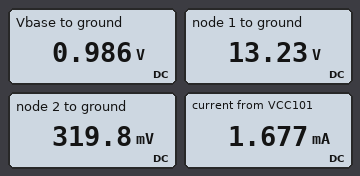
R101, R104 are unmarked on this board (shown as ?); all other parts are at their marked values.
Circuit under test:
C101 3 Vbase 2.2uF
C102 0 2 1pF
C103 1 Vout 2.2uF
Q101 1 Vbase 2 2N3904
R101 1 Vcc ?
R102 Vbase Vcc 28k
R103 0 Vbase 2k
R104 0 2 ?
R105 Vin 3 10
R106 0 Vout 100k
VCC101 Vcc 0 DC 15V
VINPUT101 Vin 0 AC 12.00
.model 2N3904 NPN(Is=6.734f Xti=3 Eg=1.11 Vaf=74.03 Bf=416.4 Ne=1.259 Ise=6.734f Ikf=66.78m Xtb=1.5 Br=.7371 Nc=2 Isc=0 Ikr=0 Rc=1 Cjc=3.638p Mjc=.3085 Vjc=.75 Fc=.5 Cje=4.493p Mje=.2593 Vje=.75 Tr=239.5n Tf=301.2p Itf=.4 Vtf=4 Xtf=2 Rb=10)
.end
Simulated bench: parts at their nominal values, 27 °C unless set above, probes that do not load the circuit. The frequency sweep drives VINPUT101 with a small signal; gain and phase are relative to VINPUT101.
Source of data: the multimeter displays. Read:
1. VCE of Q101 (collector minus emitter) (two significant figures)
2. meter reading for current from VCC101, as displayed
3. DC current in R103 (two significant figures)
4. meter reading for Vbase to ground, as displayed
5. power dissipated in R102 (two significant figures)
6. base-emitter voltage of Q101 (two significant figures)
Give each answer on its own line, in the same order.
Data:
13 V
1.677 mA
490 µA
0.986 V
7.0 mW
670 mV
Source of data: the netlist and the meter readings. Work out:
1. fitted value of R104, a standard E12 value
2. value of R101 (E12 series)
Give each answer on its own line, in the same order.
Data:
270 Ω
1.5 kΩ
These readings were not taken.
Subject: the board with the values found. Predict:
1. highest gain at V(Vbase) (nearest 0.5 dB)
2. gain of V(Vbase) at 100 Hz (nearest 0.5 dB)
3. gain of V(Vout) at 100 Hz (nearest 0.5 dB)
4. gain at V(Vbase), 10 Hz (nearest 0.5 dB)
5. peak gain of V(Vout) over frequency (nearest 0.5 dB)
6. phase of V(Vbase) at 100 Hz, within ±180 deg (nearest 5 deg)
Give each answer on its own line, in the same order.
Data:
0 dB
-0.5 dB
13.5 dB
-12.5 dB
14.0 dB
20 deg
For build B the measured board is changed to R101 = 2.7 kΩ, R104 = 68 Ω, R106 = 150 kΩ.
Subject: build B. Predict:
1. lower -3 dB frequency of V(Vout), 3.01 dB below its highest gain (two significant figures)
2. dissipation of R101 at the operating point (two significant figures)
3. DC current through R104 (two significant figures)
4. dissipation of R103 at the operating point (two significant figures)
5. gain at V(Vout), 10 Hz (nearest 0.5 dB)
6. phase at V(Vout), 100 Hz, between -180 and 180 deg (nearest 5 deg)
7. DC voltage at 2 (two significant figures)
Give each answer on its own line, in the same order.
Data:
45 Hz
38 mW
3.8 mA
460 µW
17.5 dB
-155 deg
260 mV
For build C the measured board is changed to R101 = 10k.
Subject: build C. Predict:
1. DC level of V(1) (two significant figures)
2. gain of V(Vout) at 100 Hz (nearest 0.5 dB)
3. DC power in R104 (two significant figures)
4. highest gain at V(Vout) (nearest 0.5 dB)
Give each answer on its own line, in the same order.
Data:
3.4 V
29.0 dB
370 µW
29.5 dB
